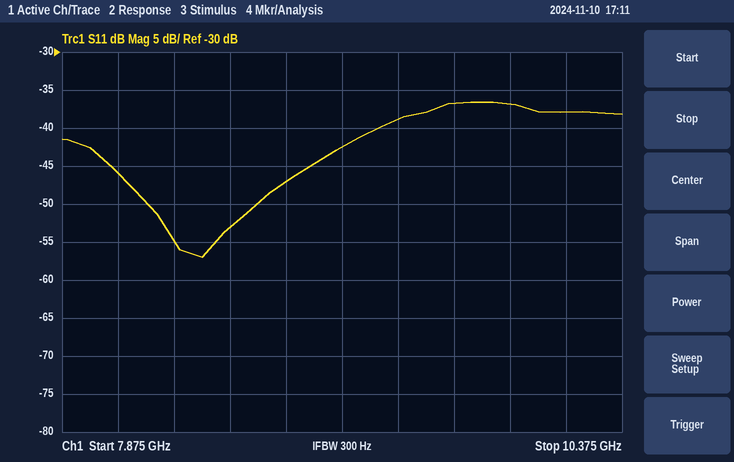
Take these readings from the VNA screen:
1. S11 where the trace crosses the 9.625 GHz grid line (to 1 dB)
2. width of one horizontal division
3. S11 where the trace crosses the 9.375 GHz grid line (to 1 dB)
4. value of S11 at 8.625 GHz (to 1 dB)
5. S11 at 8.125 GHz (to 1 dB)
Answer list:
-37 dB
250 MHz
-39 dB
-53 dB
-46 dB
